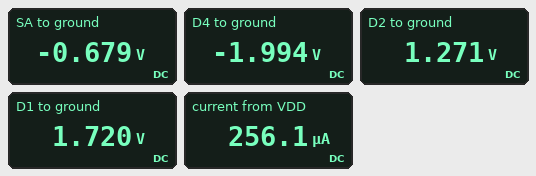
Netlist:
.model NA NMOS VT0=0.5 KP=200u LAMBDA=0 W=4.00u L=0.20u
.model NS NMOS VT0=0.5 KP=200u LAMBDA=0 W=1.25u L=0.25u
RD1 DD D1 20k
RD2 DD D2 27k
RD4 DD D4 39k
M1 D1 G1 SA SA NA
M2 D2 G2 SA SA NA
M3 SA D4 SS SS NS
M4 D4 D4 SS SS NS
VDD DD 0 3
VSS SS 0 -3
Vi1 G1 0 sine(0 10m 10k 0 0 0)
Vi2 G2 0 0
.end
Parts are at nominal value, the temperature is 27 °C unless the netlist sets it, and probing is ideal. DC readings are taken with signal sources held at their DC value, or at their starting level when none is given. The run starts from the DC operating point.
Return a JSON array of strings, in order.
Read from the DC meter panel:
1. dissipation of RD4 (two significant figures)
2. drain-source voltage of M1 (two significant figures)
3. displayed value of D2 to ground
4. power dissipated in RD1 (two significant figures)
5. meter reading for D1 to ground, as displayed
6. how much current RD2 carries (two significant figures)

["640 µW", "2.4 V", "1.271 V", "82 µW", "1.720 V", "64 µA"]
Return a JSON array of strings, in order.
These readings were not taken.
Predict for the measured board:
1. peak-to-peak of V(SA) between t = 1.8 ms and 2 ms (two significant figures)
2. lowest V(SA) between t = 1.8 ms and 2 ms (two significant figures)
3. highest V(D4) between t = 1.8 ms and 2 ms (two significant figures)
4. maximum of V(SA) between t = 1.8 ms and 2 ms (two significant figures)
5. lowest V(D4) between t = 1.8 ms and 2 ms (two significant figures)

["10 mV", "-680 mV", "-2.0 V", "-670 mV", "-2.0 V"]
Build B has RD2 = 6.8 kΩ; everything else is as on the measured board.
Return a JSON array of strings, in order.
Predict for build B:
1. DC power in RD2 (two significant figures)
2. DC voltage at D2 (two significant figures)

["28 µW", "2.6 V"]
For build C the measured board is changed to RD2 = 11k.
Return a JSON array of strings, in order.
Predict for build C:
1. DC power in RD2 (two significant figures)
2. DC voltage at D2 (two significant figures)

["45 µW", "2.3 V"]
